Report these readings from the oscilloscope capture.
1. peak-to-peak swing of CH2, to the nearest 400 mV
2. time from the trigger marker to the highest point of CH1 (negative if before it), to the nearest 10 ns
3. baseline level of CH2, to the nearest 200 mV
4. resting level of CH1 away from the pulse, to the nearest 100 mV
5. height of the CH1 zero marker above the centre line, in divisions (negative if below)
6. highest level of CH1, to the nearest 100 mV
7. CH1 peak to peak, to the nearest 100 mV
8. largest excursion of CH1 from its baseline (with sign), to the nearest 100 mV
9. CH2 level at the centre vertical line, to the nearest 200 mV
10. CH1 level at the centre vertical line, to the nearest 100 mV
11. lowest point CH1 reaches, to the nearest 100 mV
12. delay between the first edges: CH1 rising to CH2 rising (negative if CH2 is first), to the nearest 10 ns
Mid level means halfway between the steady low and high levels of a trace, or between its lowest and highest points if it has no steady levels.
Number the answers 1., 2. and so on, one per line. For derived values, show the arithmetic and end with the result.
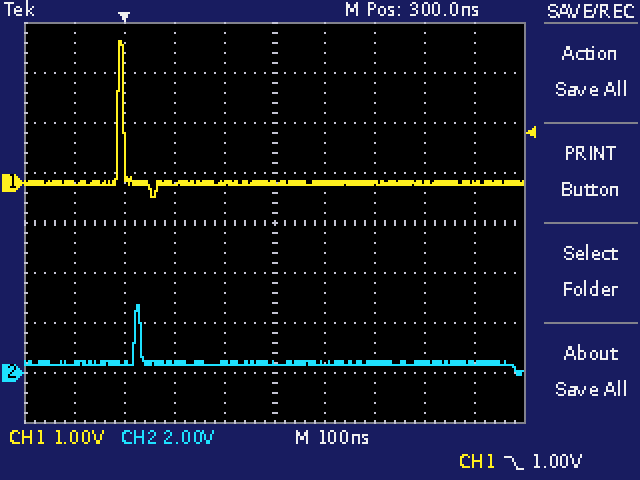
1. 2.8 V
2. -10 ns
3. 400 mV
4. 0.0 V
5. +0.8 div
6. 2.8 V
7. 2.8 V − (-300 mV) = 3.1 V
8. 2.8 V − (0.0 V) = +2.8 V
9. 400 mV
10. 0.0 V
11. -300 mV
12. +30 ns
